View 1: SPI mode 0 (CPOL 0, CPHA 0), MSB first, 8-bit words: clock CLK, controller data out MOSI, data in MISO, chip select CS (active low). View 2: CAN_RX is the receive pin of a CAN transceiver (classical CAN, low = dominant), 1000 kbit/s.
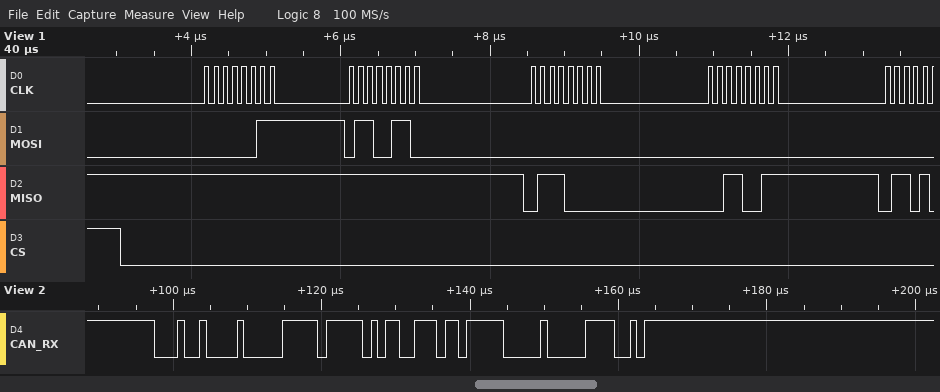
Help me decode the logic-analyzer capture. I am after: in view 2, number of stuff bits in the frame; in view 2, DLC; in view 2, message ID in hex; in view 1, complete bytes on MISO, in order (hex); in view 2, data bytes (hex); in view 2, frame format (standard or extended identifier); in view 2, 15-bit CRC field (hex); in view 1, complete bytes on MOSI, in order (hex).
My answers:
6
3
0x121
FF FF 70 33
FF 67 6F
standard
0x401C
03 66 00 00
